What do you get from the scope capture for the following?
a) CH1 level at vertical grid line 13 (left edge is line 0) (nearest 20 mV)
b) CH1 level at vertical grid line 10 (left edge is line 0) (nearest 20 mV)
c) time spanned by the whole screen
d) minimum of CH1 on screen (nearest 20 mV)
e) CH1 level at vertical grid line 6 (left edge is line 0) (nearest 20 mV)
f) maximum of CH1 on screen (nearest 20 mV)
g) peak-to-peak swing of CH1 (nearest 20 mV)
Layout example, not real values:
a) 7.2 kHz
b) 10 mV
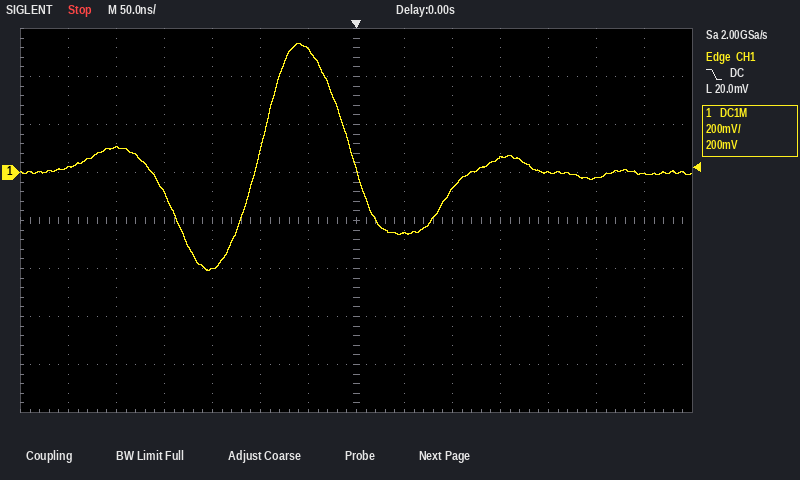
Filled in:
a) 0 mV
b) 60 mV
c) 700 ns
d) -400 mV
e) 520 mV
f) 540 mV
g) 940 mV
